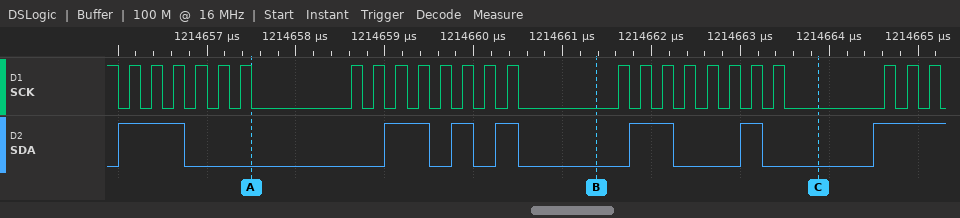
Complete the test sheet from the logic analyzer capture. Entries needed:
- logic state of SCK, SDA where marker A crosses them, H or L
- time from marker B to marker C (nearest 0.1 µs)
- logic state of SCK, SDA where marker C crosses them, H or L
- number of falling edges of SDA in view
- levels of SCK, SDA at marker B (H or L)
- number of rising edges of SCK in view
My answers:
SCK=L, SDA=L
2.5 µs
SCK=L, SDA=L
6
SCK=L, SDA=L
25
